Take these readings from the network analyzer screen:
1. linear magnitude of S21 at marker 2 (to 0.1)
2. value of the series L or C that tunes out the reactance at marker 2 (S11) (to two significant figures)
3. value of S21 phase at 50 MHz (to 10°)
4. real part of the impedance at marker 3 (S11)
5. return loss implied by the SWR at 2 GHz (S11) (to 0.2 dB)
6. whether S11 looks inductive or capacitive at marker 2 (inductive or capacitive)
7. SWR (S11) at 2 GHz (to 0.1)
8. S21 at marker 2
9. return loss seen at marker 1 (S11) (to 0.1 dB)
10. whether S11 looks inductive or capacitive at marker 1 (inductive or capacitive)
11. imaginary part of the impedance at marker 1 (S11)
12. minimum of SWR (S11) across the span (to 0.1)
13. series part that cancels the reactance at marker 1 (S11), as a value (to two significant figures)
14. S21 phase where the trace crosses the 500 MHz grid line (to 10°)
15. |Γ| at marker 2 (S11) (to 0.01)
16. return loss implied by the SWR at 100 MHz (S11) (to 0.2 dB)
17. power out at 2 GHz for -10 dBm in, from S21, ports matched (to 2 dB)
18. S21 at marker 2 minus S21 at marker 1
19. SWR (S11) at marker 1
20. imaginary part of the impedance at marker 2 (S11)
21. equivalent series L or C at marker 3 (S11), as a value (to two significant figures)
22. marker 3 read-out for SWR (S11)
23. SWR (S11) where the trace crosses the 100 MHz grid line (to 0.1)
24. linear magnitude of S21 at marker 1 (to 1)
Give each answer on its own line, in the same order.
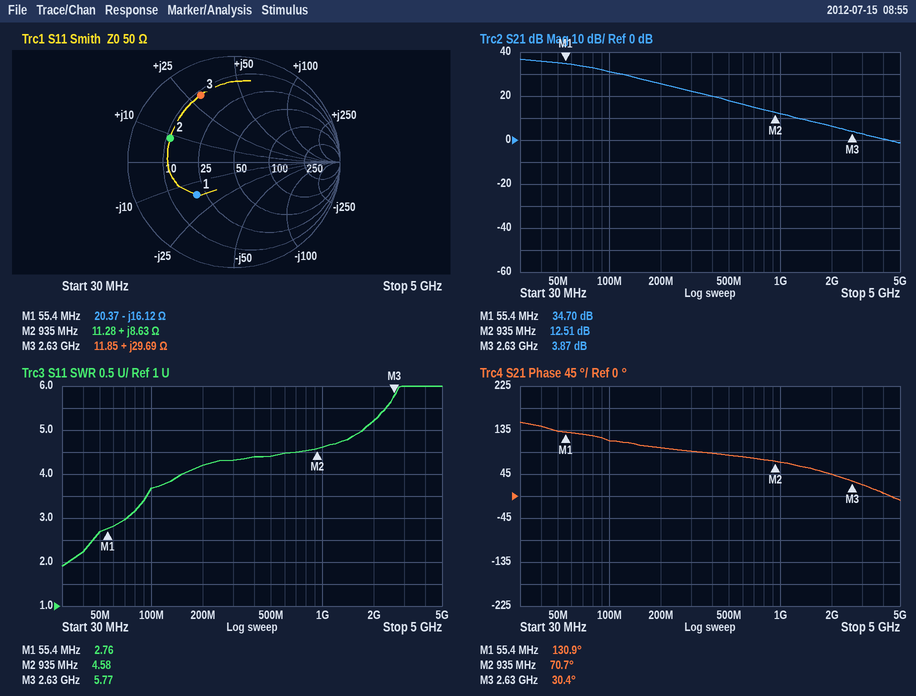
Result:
4.2
20 pF
130°
11.85 Ω
3.4 dB
inductive
5.2
12.51 dB
6.6 dB
capacitive
-16.12 Ω
1.9
46 nH
80°
0.64
4.8 dB
-4 dBm
-22.19 dB
2.76
+8.63 Ω
1.8 nH
5.77
3.7
54
